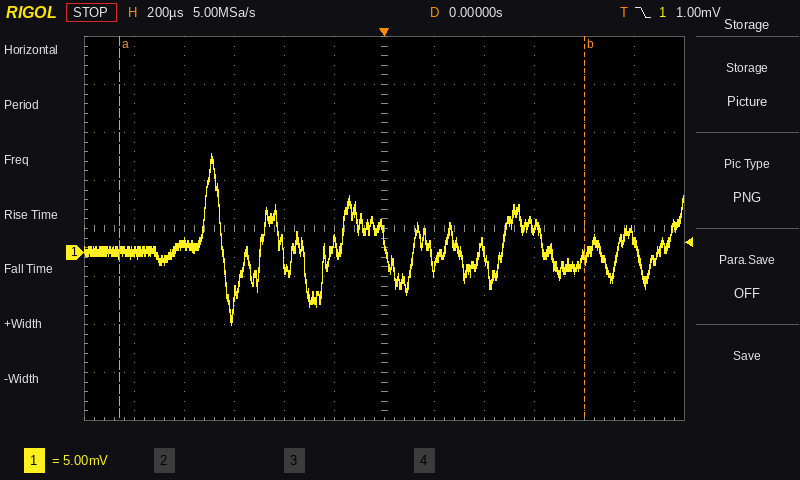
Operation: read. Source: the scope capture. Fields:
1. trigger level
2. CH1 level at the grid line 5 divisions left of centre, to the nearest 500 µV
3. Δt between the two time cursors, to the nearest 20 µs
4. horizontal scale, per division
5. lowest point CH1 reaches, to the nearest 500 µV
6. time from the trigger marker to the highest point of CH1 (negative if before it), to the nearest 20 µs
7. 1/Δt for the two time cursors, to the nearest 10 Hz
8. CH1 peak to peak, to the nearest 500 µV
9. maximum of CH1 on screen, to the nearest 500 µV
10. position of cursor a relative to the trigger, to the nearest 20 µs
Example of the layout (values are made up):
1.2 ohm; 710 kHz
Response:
1.00 mV; 0.0 mV; 1.86 ms; 200 µs; -7.5 mV; -680 µs; 540 Hz; 18.0 mV; 10.5 mV; -1.06 ms
